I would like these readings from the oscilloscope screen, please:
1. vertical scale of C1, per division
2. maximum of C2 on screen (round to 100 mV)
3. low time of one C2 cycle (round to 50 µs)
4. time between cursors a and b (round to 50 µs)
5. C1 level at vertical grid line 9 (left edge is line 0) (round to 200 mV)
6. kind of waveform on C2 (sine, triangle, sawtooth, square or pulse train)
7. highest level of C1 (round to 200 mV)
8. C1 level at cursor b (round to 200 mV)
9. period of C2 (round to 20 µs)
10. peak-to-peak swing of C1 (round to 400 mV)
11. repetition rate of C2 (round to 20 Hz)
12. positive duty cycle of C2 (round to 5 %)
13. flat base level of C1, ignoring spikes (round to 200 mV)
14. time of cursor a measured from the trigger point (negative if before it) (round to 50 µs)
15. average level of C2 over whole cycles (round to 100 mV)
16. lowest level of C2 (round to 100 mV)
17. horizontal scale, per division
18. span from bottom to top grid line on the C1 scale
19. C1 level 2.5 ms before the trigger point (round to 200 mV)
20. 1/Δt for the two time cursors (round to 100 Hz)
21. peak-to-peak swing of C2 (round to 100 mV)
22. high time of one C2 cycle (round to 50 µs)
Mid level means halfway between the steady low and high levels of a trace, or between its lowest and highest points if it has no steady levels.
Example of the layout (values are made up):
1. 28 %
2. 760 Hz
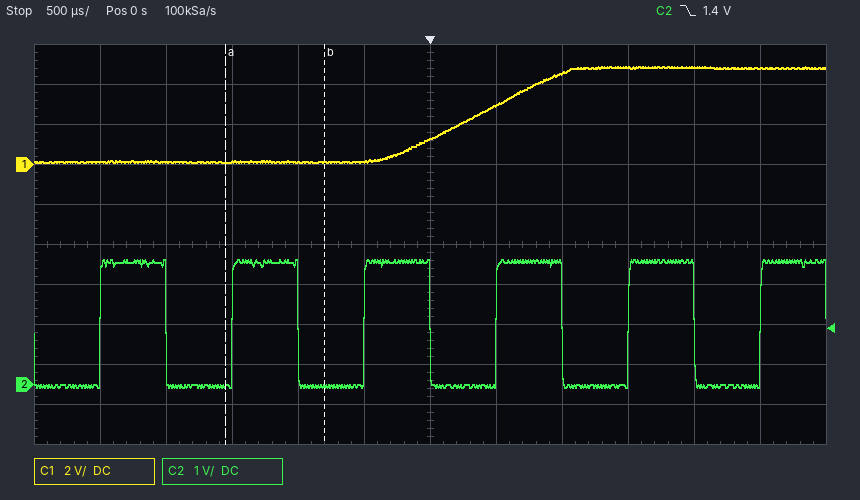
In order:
1. 2 V
2. 3.1 V
3. 500 µs
4. 750 µs
5. 4.8 V
6. square
7. 4.8 V
8. 200 mV
9. 1.00 ms
10. 4.8 V
11. 1.00 kHz
12. 50 %
13. 200 mV
14. -1.55 ms
15. 1.5 V
16. -100 mV
17. 500 µs
18. 20 V
19. 200 mV
20. 1.3 kHz
21. 3.2 V
22. 500 µs
